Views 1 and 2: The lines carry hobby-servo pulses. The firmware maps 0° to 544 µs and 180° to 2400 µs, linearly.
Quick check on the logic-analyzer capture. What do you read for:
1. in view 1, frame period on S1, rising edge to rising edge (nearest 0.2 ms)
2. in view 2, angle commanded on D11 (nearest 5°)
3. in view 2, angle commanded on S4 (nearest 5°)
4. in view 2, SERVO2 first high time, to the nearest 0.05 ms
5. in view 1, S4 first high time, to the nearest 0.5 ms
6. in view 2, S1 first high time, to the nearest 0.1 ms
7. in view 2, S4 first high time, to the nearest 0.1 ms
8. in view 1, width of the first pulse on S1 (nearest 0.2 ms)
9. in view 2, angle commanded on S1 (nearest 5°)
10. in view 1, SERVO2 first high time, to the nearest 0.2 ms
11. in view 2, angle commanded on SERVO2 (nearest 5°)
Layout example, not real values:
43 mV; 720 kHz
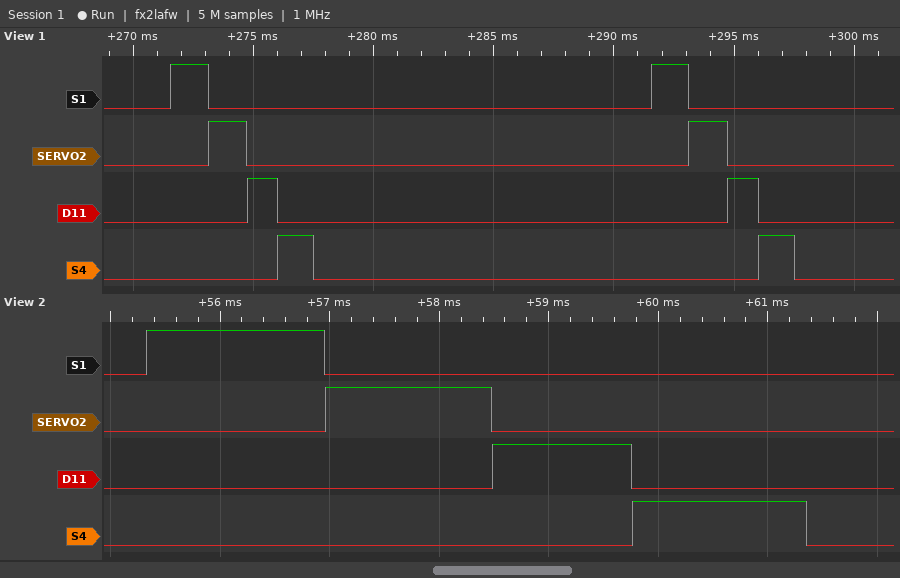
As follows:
20.0 ms; 70°; 100°; 1.50 ms; 1.5 ms; 1.6 ms; 1.6 ms; 1.6 ms; 105°; 1.6 ms; 95°
